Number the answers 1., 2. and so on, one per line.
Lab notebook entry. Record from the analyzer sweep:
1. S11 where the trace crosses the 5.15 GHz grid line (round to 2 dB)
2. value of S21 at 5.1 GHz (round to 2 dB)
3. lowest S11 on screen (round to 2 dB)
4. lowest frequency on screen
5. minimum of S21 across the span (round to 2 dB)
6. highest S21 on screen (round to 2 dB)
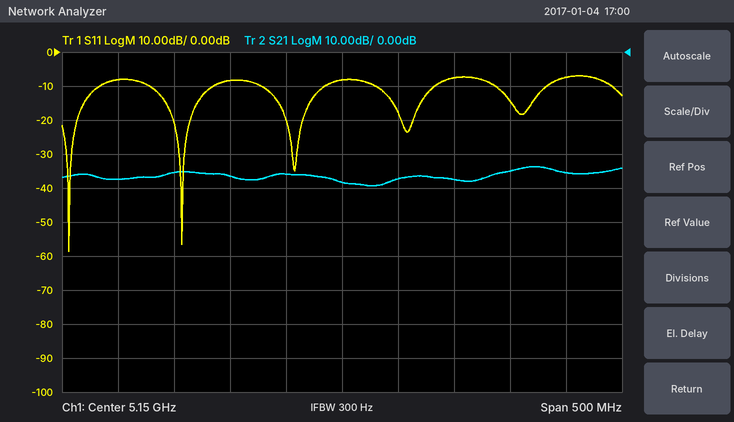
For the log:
1. -8 dB
2. -36 dB
3. -58 dB
4. 4.9 GHz
5. -40 dB
6. -34 dB
